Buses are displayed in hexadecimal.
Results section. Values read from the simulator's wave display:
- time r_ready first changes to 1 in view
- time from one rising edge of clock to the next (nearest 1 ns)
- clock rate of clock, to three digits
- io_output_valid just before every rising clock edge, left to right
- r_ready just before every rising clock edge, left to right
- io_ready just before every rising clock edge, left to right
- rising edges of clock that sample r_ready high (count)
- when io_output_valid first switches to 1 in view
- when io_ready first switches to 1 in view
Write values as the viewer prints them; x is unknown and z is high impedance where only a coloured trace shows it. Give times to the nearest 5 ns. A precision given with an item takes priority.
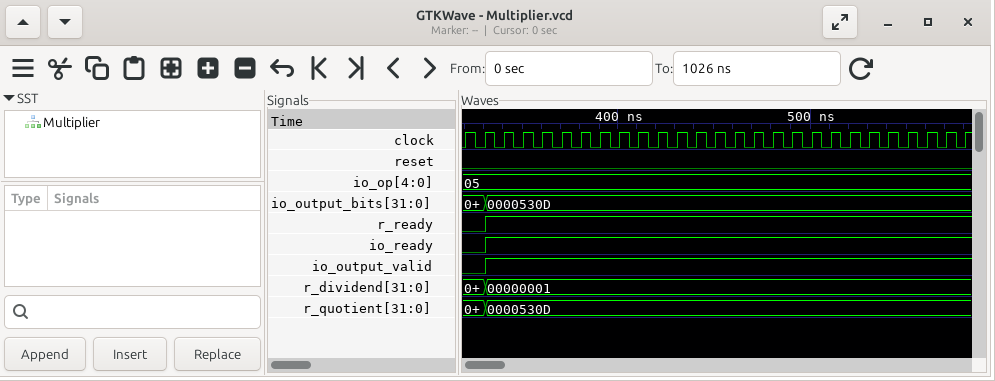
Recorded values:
330 ns
10 ns
100 MHz
0 0 1 1 1 1 1 1 1 1 1 1 1 1 1 1 1 1 1 1 1 1 1 1 1 1 1
0 0 1 1 1 1 1 1 1 1 1 1 1 1 1 1 1 1 1 1 1 1 1 1 1 1 1
0 0 1 1 1 1 1 1 1 1 1 1 1 1 1 1 1 1 1 1 1 1 1 1 1 1 1
25
330 ns
330 ns
